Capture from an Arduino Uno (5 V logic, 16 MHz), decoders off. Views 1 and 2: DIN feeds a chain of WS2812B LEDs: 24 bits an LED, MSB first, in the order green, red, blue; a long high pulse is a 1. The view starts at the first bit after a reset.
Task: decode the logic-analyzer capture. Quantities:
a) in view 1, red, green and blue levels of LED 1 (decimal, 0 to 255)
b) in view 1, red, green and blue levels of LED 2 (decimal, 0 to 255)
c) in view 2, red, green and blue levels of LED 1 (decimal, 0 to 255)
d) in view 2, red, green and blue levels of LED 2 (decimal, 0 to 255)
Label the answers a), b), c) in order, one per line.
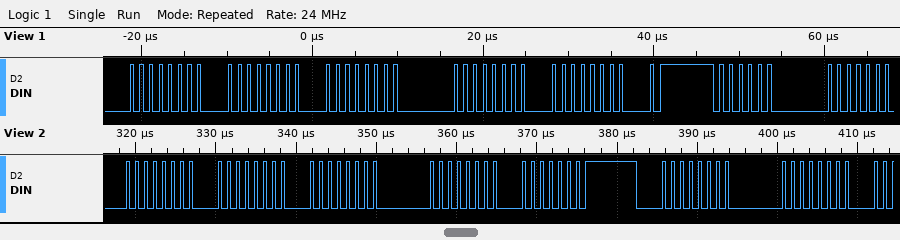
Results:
a) 0, 0, 0
b) 0, 0, 64
c) 0, 0, 0
d) 1, 0, 0
